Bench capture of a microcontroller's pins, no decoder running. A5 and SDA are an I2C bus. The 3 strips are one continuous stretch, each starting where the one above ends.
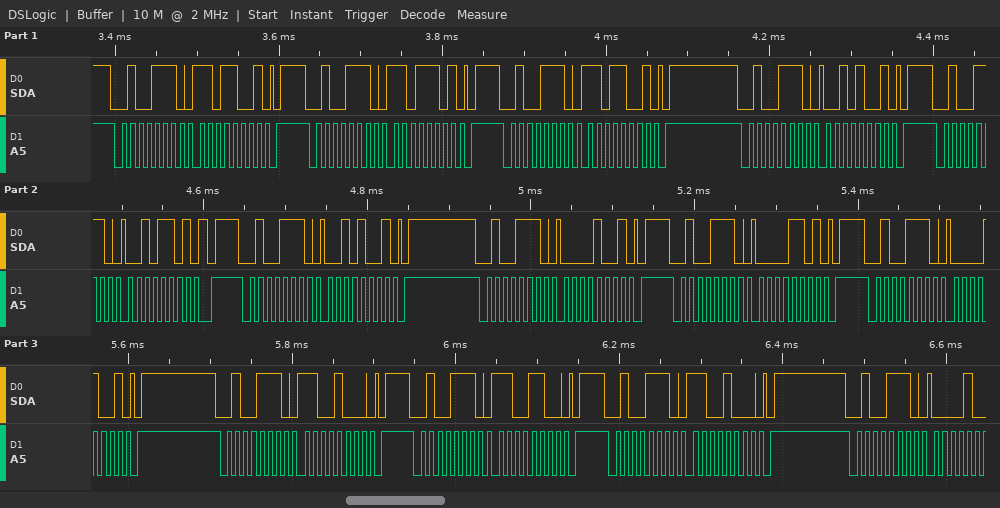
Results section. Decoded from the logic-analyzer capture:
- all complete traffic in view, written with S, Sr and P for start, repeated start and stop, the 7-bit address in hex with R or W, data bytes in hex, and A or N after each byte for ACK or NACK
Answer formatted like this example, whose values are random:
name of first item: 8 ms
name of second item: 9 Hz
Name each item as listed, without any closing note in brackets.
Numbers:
all complete traffic in view, written with S, Sr and P for start, repeated start and stop, the 7-bit address in hex with R or W, data bytes in hex, and A or N after each byte for ACK or NACK: S 27W A D9 A P S 27W A DD A P S 27W A D9 A P S 27W A 29 A P S 27W A 2D A P S 27W A 29 A P S 27W A 09 A P S 27W A 0D A P S 27W A 09 A P S 27W A C8 A P S 27W A CC A P S 27W A C8 A P S 27W A
